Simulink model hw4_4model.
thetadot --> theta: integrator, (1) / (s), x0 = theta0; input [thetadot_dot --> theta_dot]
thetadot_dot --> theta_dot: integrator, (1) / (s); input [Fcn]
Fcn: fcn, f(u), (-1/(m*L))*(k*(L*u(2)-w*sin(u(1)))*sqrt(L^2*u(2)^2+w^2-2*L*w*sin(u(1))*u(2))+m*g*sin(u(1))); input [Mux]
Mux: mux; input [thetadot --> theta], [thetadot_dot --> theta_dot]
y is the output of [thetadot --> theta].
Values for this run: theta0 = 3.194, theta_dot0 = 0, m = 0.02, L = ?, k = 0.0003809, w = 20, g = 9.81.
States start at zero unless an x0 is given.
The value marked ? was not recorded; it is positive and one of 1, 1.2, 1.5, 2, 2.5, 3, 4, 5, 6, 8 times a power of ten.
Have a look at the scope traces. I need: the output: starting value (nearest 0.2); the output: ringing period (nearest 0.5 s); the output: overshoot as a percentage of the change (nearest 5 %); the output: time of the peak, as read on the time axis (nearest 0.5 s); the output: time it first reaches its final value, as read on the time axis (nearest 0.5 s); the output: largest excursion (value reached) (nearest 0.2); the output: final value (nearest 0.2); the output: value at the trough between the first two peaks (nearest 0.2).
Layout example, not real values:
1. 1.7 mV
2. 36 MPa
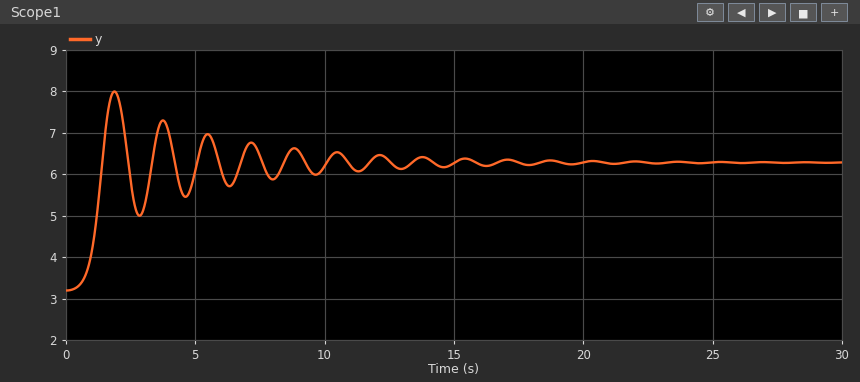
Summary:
1. 3.2
2. 2.0 s
3. 55 %
4. 2.0 s
5. 1.5 s
6. 8.0
7. 6.2
8. 5.0
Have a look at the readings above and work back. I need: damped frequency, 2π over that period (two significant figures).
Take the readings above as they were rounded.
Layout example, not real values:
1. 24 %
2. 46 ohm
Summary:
1. 3.1 rad/s
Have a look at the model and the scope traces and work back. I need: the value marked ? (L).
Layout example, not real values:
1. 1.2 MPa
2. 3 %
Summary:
1. 0.15
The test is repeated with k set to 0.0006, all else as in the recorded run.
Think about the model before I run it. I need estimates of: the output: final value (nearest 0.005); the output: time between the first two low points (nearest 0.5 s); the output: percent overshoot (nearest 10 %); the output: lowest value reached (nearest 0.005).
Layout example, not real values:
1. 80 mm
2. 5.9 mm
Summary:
1. 3.140
2. 1.5 s
3. 80 %
4. 3.100
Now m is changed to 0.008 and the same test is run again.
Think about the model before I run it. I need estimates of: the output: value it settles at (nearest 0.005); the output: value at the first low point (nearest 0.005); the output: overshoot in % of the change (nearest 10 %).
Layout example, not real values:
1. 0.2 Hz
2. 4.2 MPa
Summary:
1. 3.140
2. 3.100
3. 80 %
